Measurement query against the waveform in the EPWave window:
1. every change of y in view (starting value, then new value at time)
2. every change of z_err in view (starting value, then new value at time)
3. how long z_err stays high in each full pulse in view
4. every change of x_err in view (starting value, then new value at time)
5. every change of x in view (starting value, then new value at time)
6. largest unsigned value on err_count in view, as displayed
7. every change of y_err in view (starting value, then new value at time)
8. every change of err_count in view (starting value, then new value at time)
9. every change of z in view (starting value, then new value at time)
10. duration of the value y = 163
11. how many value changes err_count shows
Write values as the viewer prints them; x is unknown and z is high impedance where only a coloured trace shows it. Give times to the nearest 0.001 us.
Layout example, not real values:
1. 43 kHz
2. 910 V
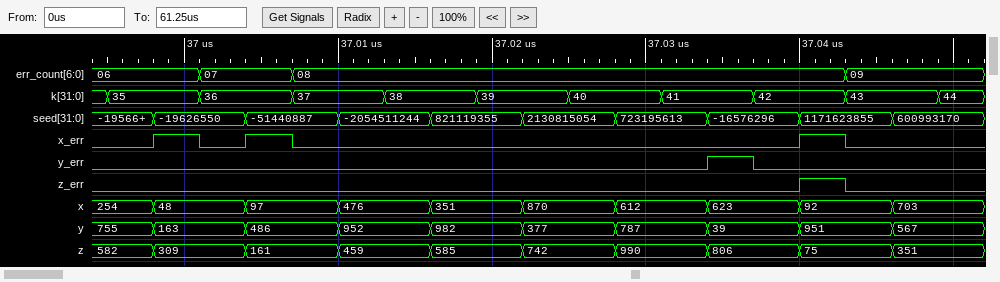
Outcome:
1. 755, 163 at 36.998 us, 486 at 37.004 us, 952 at 37.01 us, 982 at 37.016 us, 377 at 37.022 us, 787 at 37.028 us, 39 at 37.034 us, 951 at 37.04 us, 567 at 37.046 us
2. 0, 1 at 37.04 us, 0 at 37.043 us
3. 0.003 us
4. 0, 1 at 36.998 us, 0 at 37.001 us, 1 at 37.004 us, 0 at 37.007 us, 1 at 37.04 us, 0 at 37.043 us
5. 254, 48 at 36.998 us, 97 at 37.004 us, 476 at 37.01 us, 351 at 37.016 us, 870 at 37.022 us, 612 at 37.028 us, 623 at 37.034 us, 92 at 37.04 us, 703 at 37.046 us
6. 09
7. 0, 1 at 37.034 us, 0 at 37.037 us
8. 06, 07 at 37.001 us, 08 at 37.007 us, 09 at 37.043 us
9. 582, 309 at 36.998 us, 161 at 37.004 us, 459 at 37.01 us, 585 at 37.016 us, 742 at 37.022 us, 990 at 37.028 us, 806 at 37.034 us, 75 at 37.04 us, 351 at 37.046 us
10. 0.006 us
11. 3
